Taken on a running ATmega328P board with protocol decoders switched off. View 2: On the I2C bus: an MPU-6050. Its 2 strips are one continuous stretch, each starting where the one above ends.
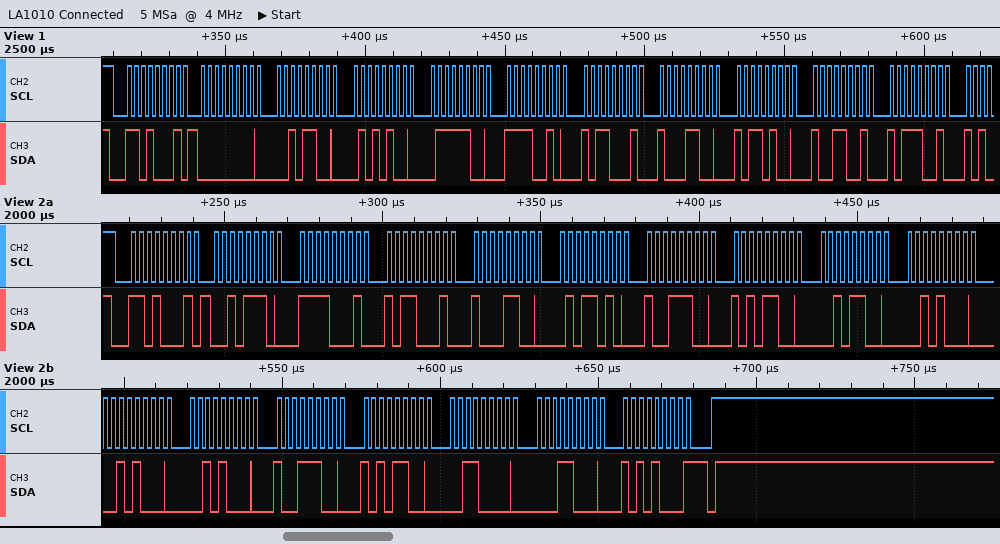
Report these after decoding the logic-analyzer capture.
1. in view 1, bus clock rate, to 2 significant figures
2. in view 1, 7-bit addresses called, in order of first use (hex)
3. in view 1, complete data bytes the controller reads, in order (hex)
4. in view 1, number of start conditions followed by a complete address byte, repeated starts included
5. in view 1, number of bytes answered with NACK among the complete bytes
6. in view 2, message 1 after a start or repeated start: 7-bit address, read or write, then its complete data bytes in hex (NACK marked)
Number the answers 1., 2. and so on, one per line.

1. 400 kHz
2. 0x68
3. 00 2C 54 7C F2 B1 8C B4 99 B9
4. 1
5. 0
6. 0x68 read: 2E F1 B1 8C 5A 9C AC 2C 28 28 28 9C AC 30 18 A8 NACK
